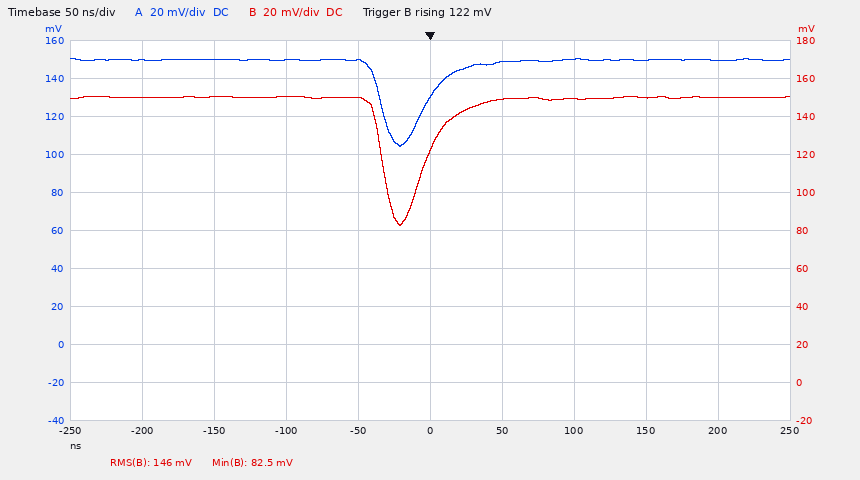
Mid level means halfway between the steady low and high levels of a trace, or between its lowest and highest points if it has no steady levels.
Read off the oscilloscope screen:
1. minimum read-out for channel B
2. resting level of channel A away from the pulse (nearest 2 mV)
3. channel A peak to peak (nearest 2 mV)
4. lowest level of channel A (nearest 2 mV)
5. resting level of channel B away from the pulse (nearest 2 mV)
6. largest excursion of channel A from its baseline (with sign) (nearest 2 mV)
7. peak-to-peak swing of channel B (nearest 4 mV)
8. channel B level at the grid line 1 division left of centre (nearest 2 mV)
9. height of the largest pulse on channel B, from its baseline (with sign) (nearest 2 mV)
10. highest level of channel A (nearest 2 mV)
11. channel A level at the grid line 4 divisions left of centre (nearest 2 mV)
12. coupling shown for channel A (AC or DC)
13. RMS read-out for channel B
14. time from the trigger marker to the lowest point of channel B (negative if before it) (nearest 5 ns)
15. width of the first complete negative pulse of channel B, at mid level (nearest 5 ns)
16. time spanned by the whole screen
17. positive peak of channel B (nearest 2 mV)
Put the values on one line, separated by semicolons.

82.5 mV; 150 mV; 46 mV; 104 mV; 150 mV; -46 mV; 68 mV; 150 mV; -68 mV; 150 mV; 150 mV; DC; 146 mV; -20 ns; 30 ns; 500 ns; 150 mV
